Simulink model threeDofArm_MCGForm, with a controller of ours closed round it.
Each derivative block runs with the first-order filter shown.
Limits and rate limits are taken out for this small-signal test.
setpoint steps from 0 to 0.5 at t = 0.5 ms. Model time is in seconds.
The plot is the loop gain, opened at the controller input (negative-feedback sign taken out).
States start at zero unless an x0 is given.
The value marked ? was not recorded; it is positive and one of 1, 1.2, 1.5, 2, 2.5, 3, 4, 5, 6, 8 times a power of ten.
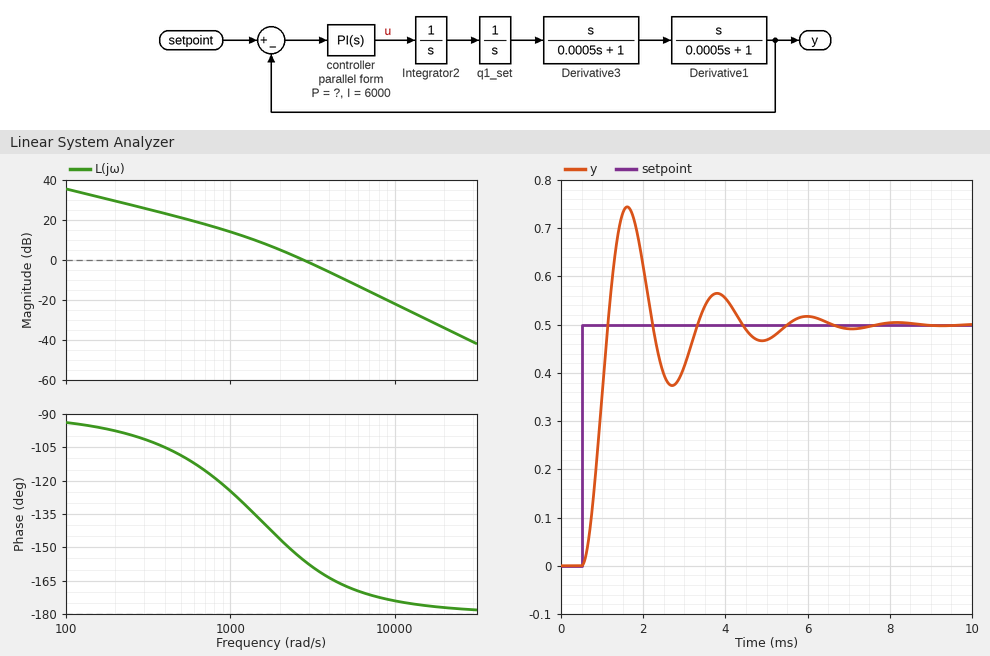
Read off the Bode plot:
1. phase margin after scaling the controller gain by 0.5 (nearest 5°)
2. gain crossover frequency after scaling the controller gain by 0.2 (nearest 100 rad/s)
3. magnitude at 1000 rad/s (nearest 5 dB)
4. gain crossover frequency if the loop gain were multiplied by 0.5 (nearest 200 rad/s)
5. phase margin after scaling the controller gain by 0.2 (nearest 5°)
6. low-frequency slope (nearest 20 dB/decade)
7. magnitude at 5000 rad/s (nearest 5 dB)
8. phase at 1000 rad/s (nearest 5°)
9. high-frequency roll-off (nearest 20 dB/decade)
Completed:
35°
1000 rad/s
15 dB
1800 rad/s
55°
-20 dB/decade
-10 dB
-125°
-40 dB/decade
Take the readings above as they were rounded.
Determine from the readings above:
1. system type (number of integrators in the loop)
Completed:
1
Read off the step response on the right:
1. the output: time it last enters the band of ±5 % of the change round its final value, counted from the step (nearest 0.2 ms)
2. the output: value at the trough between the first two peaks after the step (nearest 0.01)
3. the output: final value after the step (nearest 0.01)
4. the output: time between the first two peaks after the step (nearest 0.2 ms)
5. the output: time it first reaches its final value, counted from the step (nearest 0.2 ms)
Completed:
4.6 ms
0.37
0.50
2.2 ms
0.6 ms
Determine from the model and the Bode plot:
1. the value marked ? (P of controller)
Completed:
2
